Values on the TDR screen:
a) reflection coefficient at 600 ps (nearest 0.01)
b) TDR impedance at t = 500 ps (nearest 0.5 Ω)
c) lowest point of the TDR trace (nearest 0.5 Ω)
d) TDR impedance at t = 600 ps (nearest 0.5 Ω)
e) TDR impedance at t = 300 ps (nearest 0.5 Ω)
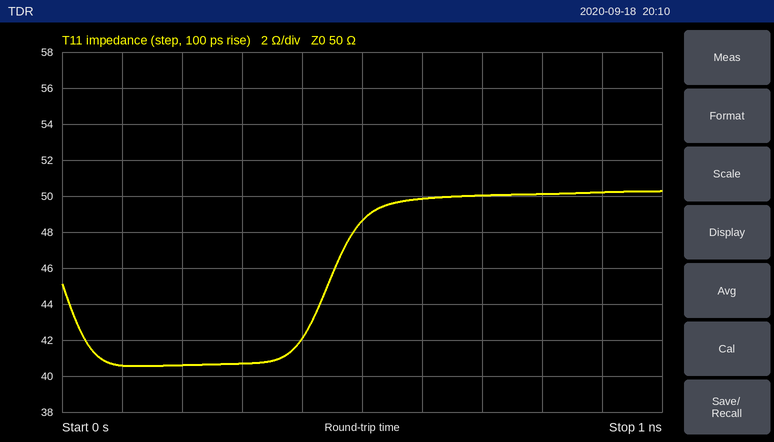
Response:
0.00
48.5 Ω
40.5 Ω
50.0 Ω
40.5 Ω
